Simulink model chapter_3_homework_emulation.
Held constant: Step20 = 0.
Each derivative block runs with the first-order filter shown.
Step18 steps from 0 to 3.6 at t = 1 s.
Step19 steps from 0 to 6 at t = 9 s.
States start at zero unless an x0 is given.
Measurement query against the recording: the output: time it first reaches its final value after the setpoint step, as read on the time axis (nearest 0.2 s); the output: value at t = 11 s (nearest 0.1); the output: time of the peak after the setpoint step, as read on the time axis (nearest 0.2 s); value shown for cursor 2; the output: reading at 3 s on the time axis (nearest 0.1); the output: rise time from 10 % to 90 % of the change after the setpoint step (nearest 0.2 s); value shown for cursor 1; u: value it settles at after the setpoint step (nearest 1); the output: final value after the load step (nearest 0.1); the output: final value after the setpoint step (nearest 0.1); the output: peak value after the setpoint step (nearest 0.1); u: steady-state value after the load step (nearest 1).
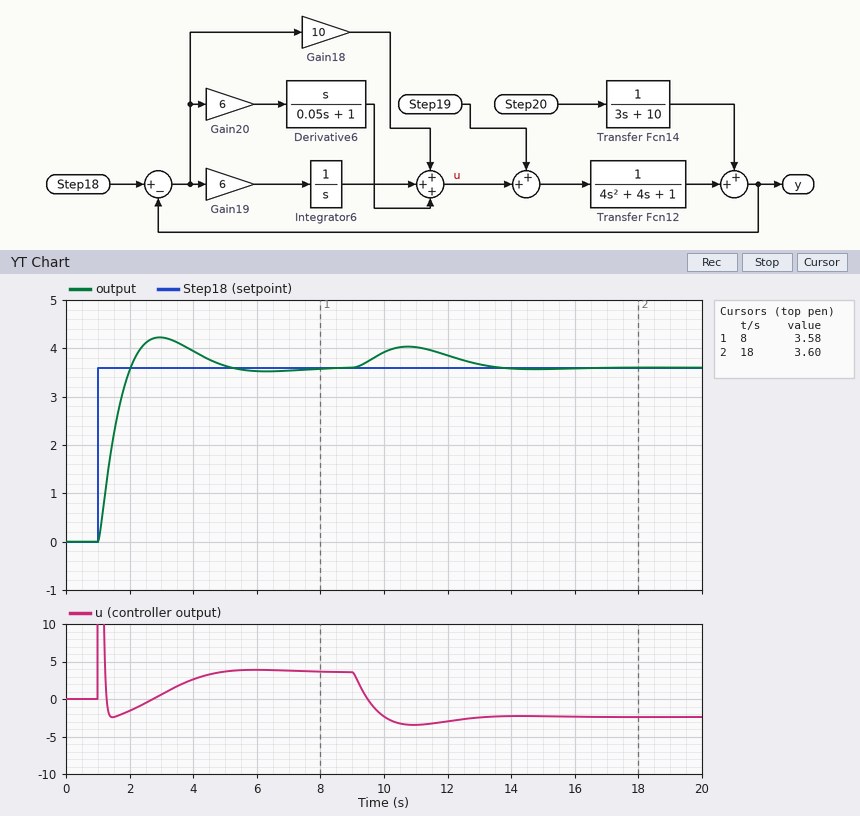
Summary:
2.0 s
4.0
3.0 s
3.60
4.2
0.8 s
3.58
4
3.6
3.6
4.2
-2
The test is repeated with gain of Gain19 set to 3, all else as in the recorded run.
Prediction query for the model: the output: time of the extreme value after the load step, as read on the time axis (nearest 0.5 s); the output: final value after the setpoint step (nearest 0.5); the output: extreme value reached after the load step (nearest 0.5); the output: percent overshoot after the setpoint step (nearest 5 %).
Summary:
11.0 s
3.5
4.0
10 %
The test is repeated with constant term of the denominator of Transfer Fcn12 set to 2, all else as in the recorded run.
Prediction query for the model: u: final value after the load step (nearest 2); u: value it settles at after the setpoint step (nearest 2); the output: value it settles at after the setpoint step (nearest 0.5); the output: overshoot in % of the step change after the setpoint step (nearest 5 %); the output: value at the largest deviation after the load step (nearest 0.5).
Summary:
2
8
3.5
10 %
4.0
